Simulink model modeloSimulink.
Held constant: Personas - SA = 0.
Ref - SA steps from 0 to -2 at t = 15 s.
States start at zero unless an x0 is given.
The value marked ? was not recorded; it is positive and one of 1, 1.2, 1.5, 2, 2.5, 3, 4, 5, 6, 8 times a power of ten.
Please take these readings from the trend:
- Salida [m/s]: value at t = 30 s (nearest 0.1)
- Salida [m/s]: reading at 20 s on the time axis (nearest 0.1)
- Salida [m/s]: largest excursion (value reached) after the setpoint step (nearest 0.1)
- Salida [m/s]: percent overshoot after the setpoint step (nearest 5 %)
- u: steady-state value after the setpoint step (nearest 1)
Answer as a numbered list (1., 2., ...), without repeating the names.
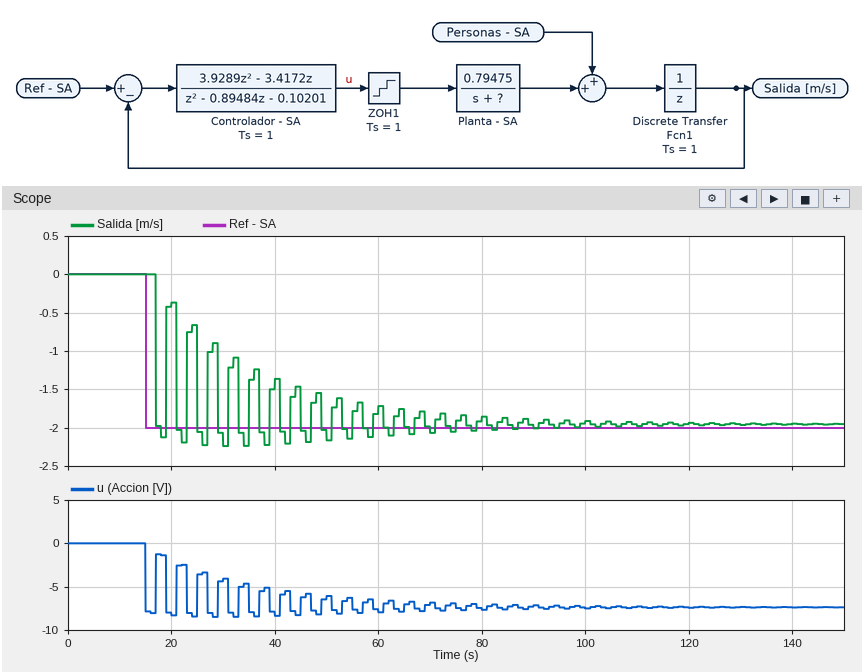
1. -2.2
2. -0.4
3. -2.2
4. 15 %
5. -7
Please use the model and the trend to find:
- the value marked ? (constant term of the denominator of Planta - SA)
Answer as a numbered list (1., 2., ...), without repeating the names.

1. 3
